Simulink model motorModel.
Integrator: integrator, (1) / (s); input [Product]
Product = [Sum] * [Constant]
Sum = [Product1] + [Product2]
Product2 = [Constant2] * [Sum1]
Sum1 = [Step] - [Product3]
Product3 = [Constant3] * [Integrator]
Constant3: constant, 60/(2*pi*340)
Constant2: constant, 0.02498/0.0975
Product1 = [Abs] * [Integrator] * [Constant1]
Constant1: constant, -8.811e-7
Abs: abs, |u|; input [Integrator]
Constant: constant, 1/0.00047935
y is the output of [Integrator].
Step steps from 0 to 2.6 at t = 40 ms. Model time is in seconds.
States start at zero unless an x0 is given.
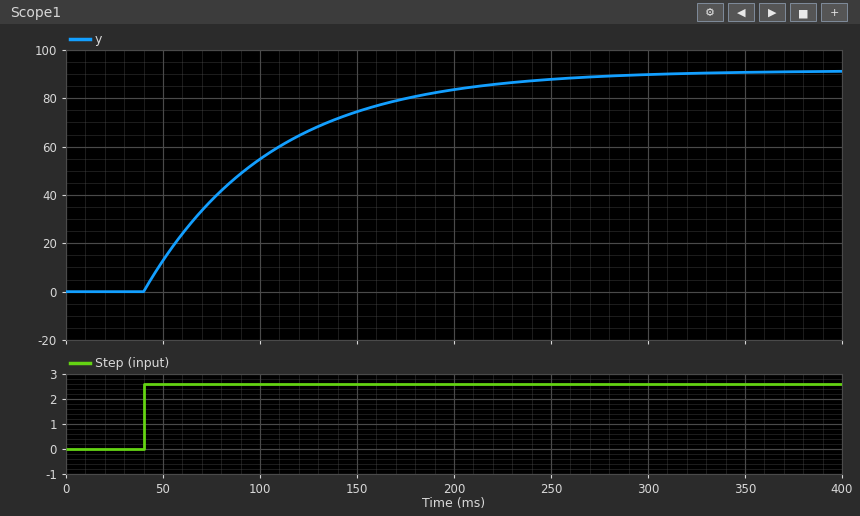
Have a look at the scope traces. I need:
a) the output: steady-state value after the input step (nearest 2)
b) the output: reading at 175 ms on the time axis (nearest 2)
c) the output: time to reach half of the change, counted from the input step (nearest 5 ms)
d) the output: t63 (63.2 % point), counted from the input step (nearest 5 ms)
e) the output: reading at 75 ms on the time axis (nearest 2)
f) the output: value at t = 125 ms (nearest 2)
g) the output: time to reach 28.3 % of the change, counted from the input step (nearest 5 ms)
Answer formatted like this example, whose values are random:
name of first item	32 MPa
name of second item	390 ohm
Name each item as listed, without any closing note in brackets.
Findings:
the output: steady-state value after the input step	92
the output: reading at 175 ms on the time axis	80
the output: time to reach half of the change, counted from the input step	45 ms
the output: t63 (63.2 % point), counted from the input step	65 ms
the output: reading at 75 ms on the time axis	38
the output: value at t = 125 ms	66
the output: time to reach 28.3 % of the change, counted from the input step	20 ms
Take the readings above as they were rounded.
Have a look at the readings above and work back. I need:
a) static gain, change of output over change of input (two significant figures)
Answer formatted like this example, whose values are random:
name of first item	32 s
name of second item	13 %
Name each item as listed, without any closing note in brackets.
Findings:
static gain, change of output over change of input	35
